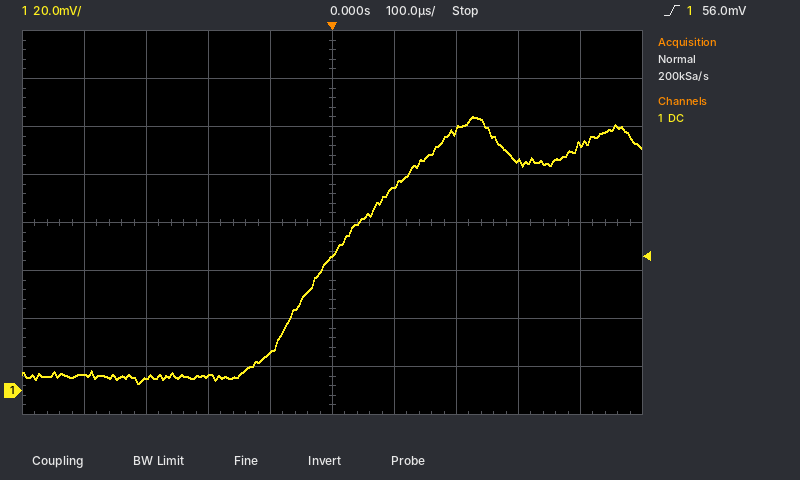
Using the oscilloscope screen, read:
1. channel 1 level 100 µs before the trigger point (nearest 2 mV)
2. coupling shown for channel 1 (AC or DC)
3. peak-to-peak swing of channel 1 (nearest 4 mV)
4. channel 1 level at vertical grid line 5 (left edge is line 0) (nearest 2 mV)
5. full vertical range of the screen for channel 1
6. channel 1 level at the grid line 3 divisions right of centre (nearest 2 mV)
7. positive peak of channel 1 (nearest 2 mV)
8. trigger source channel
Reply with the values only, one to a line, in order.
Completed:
16 mV
DC
112 mV
56 mV
160 mV
96 mV
114 mV
channel 1
